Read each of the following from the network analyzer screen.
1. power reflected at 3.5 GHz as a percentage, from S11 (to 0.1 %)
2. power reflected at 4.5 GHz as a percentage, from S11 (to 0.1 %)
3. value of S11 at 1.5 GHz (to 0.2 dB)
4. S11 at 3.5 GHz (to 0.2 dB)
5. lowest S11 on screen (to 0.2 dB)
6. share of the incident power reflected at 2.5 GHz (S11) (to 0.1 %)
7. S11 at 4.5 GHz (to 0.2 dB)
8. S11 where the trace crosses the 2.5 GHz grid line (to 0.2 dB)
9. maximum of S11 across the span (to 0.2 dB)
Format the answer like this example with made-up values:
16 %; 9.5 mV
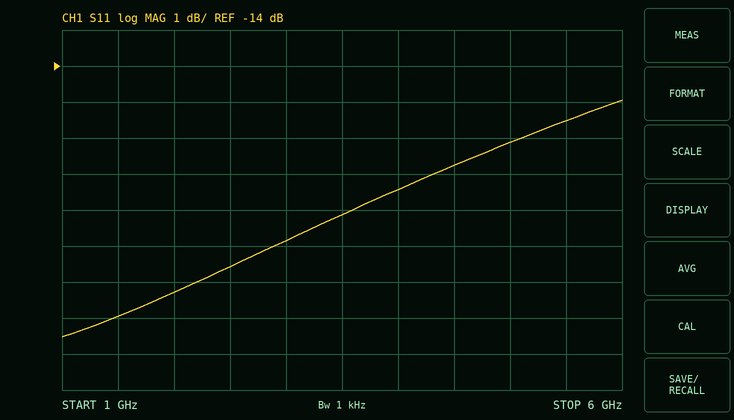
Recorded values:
1.5 %; 2.1 %; -21.0 dB; -18.2 dB; -21.6 dB; 1.1 %; -16.8 dB; -19.6 dB; -15.0 dB
